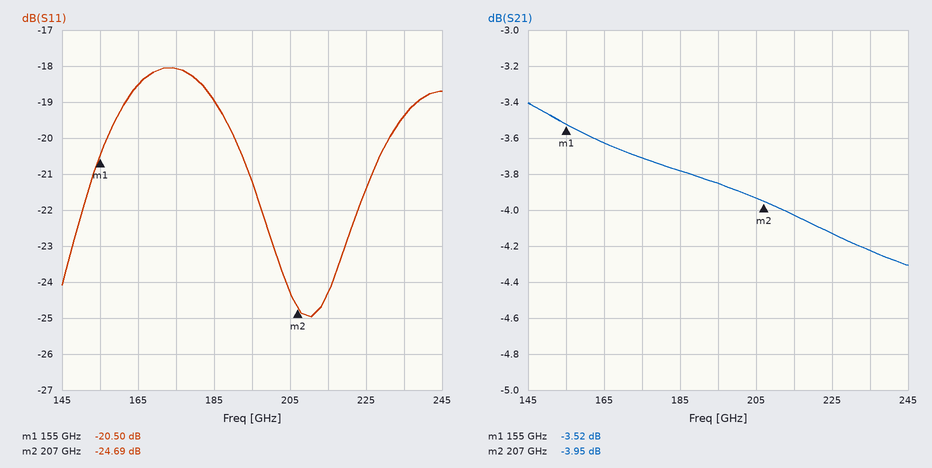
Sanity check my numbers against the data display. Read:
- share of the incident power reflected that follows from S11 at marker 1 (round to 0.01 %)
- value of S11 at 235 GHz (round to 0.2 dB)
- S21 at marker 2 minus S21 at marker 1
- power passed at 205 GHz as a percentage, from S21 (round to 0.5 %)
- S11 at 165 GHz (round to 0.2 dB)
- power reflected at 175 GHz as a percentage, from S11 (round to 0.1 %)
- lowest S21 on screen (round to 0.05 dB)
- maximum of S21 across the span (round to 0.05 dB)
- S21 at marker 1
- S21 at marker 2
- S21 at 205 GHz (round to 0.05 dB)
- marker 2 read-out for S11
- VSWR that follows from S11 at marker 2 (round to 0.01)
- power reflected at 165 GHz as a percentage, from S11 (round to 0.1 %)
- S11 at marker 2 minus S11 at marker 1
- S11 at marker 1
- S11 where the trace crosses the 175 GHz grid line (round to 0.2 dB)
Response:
0.89 %
-19.4 dB
-0.43 dB
40.5 %
-18.6 dB
1.6 %
-4.30 dB
-3.40 dB
-3.52 dB
-3.95 dB
-3.95 dB
-24.69 dB
1.12
1.4 %
-4.19 dB
-20.50 dB
-18.0 dB
